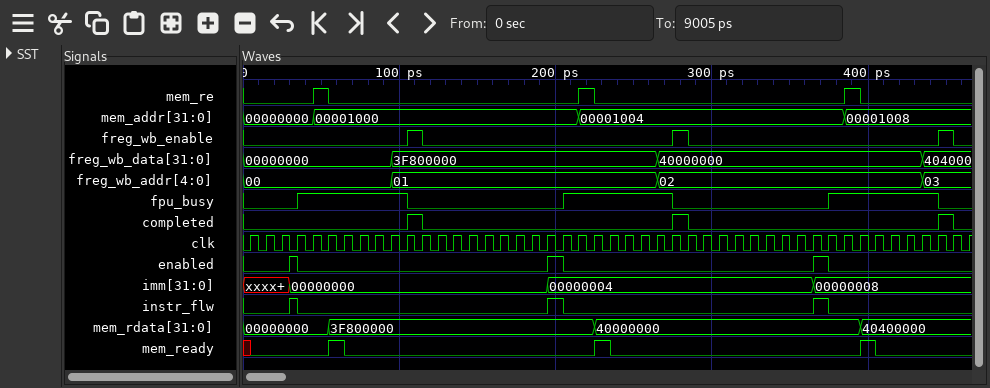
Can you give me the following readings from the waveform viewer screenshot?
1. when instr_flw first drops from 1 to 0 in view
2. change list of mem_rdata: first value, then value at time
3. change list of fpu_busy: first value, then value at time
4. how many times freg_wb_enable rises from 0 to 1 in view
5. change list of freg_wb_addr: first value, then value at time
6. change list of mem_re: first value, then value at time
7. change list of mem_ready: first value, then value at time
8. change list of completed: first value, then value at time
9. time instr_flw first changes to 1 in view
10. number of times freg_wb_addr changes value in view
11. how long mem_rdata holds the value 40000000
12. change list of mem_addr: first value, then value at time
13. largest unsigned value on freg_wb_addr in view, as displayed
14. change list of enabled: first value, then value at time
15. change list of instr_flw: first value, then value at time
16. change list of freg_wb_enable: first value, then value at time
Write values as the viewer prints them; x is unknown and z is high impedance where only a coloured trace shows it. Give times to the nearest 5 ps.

35 ps
00000000, 3F800000 at 55 ps, 40000000 at 225 ps, 40400000 at 395 ps
0, 1 at 35 ps, 0 at 105 ps, 1 at 205 ps, 0 at 275 ps, 1 at 375 ps, 0 at 445 ps
3
00, 01 at 95 ps, 02 at 265 ps, 03 at 435 ps
0, 1 at 45 ps, 0 at 55 ps, 1 at 215 ps, 0 at 225 ps, 1 at 385 ps, 0 at 395 ps
x, 0 at 5 ps, 1 at 55 ps, 0 at 65 ps, 1 at 225 ps, 0 at 235 ps, 1 at 395 ps, 0 at 405 ps
0, 1 at 105 ps, 0 at 115 ps, 1 at 275 ps, 0 at 285 ps, 1 at 445 ps, 0 at 455 ps
30 ps
3
170 ps
00000000, 00001000 at 45 ps, 00001004 at 215 ps, 00001008 at 385 ps
03
0, 1 at 30 ps, 0 at 35 ps, 1 at 195 ps, 0 at 205 ps, 1 at 365 ps, 0 at 375 ps
0, 1 at 30 ps, 0 at 35 ps, 1 at 195 ps, 0 at 205 ps, 1 at 365 ps, 0 at 375 ps
0, 1 at 105 ps, 0 at 115 ps, 1 at 275 ps, 0 at 285 ps, 1 at 445 ps, 0 at 455 ps
